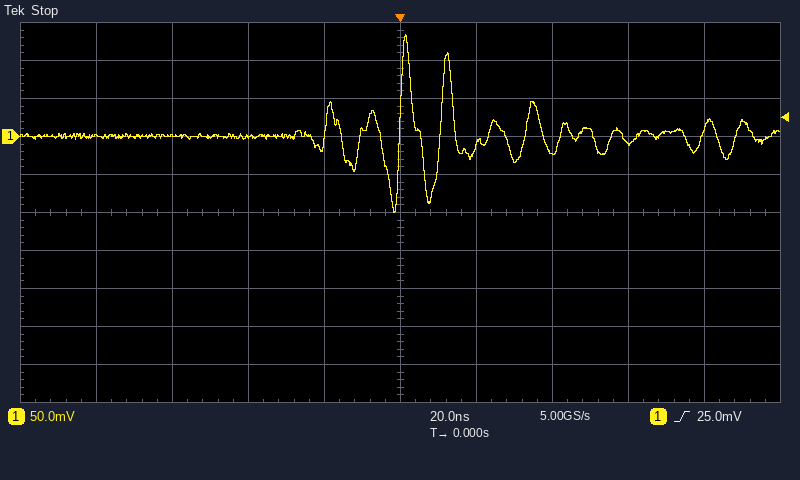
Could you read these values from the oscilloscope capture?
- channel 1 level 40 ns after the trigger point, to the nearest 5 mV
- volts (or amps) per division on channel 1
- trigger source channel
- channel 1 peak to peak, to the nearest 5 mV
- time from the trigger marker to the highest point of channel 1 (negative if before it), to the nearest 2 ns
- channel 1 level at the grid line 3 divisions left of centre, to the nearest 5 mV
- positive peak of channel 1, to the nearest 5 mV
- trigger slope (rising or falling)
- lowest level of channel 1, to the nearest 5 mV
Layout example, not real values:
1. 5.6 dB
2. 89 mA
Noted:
1. -20 mV
2. 50 mV
3. channel 1
4. 235 mV
5. +2 ns
6. 0 mV
7. 135 mV
8. rising
9. -100 mV
